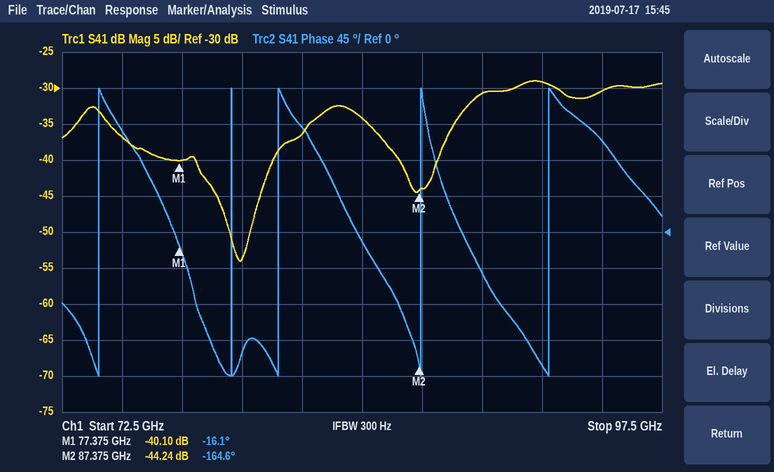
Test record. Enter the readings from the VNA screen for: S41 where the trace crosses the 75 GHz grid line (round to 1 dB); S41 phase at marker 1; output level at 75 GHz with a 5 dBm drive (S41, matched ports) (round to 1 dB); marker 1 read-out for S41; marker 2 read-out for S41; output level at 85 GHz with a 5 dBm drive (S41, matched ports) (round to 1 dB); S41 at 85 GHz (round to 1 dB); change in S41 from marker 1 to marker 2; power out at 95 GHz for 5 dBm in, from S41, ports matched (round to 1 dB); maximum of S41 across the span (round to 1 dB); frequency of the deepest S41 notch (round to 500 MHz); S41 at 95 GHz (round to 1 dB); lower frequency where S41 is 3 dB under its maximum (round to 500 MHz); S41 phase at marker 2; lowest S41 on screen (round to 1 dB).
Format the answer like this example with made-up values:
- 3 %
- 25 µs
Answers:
- -37 dB
- -16.1°
- -32 dBm
- -40.10 dB
- -44.24 dB
- -29 dBm
- -34 dB
- -4.14 dB
- -25 dBm
- -29 dB
- 80.0 GHz
- -30 dB
- 89.5 GHz
- -164.6°
- -54 dB
